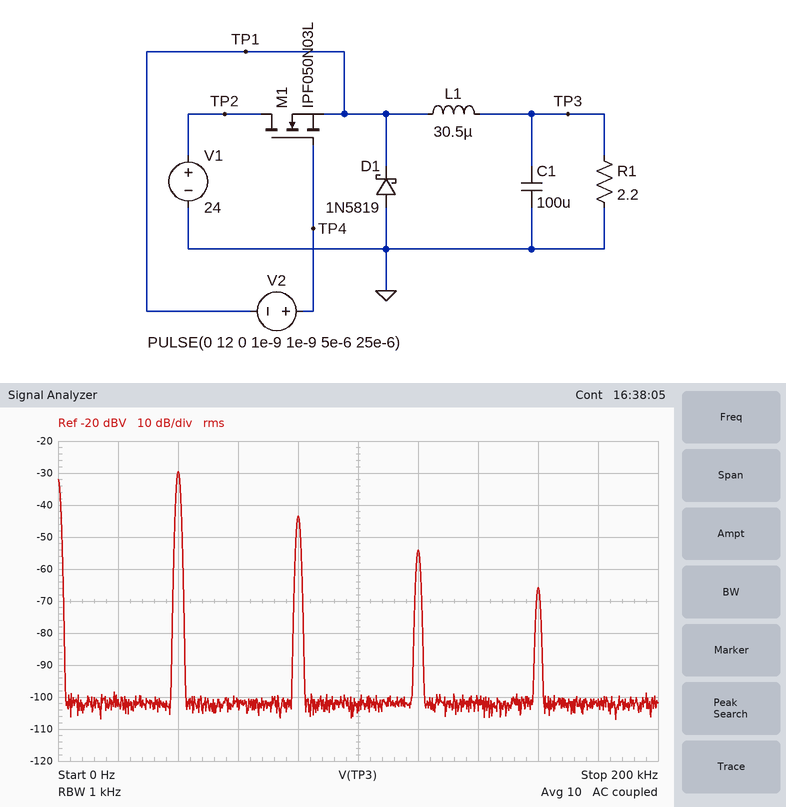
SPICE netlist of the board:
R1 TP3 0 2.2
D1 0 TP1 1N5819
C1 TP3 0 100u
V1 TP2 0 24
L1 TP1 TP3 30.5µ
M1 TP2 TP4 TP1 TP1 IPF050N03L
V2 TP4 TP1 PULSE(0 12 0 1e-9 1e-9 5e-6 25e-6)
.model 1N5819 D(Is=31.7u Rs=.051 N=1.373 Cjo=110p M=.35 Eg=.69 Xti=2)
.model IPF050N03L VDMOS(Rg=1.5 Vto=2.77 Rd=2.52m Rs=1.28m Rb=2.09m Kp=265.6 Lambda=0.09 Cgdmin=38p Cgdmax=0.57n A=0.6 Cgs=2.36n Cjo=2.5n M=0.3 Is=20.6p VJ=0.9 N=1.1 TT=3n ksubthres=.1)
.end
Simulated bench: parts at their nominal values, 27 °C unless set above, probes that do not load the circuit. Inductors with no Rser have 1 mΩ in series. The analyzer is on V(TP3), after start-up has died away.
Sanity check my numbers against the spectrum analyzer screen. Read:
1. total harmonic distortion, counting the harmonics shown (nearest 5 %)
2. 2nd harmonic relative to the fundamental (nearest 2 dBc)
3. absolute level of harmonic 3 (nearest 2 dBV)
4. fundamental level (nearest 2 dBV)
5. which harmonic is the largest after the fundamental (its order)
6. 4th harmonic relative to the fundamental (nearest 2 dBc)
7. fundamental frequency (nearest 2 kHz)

20 %
-14 dBc
-54 dBV
-30 dBV
2
-36 dBc
40 kHz
